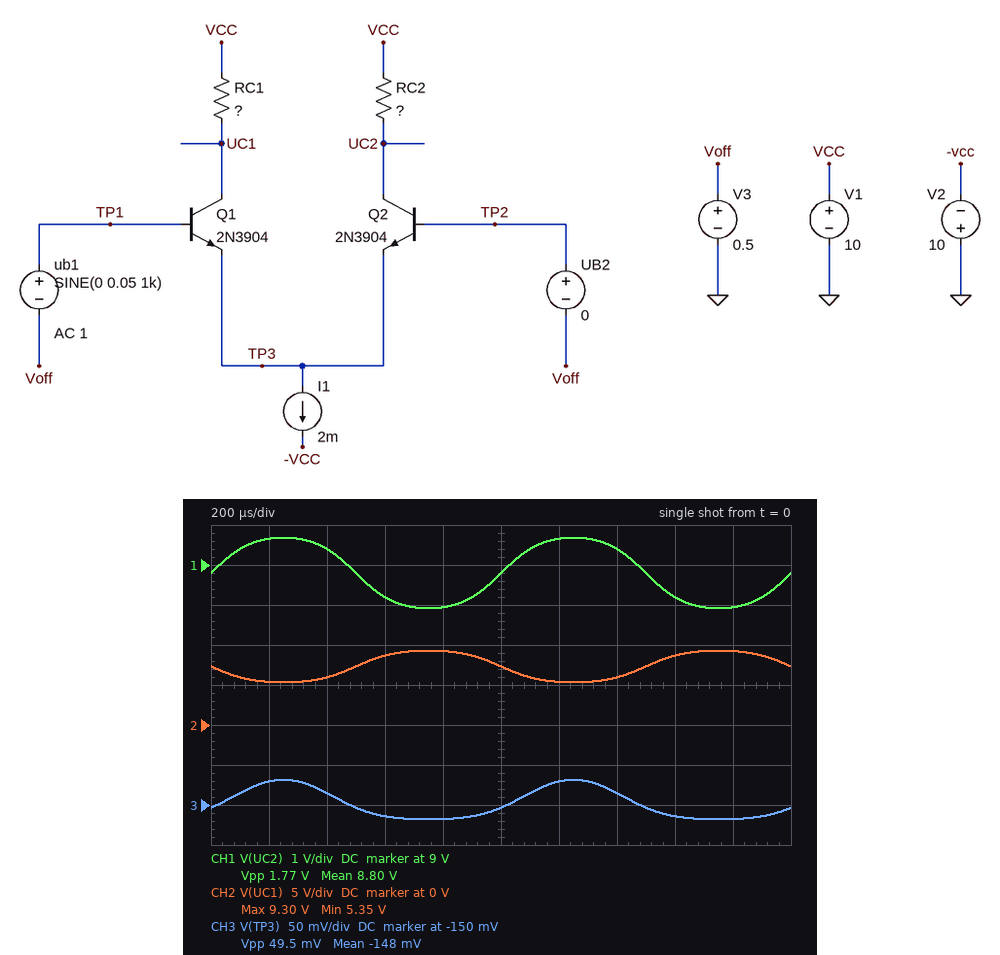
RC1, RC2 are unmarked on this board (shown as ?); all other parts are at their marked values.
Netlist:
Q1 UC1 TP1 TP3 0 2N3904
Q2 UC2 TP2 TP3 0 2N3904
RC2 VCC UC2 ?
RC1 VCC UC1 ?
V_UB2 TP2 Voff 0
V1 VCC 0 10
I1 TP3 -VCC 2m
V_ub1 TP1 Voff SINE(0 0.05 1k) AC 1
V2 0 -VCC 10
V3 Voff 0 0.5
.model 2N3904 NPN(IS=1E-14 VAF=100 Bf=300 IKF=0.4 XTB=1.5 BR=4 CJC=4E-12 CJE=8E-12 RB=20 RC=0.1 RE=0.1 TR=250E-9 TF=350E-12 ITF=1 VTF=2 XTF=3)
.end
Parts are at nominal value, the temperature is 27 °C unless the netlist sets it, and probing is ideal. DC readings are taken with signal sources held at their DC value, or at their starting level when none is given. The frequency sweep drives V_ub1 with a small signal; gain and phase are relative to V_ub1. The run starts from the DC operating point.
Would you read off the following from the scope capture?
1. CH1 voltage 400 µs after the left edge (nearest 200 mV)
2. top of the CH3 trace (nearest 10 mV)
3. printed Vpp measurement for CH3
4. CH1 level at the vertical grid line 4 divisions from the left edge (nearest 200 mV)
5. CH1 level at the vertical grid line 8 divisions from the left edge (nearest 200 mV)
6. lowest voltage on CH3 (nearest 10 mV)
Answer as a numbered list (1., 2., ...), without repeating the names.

1. 9.4 V
2. -120 mV
3. 49.5 mV
4. 8.0 V
5. 8.2 V
6. -170 mV
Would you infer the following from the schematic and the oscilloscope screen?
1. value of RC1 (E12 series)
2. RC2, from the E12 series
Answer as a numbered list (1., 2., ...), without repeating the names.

1. 2.7 kΩ
2. 1.2 kΩ
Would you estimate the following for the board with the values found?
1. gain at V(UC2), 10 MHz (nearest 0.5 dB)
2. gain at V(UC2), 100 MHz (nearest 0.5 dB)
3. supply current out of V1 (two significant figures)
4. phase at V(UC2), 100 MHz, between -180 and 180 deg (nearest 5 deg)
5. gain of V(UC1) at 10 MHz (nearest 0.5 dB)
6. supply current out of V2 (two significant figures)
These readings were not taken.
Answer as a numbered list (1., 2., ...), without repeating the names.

1. 26.5 dB
2. 18.0 dB
3. 2.0 mA
4. -75 deg
5. 33.0 dB
6. 2.0 mA
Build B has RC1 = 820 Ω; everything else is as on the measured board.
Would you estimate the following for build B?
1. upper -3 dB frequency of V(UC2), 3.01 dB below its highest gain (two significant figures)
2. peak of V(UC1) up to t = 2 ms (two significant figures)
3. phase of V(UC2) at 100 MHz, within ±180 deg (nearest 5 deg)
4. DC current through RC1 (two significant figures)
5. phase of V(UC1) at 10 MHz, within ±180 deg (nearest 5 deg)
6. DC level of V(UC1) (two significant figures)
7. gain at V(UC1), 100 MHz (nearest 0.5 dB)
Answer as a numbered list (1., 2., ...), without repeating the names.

1. 43 MHz
2. 9.8 V
3. -80 deg
4. 1.0 mA
5. 170 deg
6. 9.2 V
7. 17.5 dB
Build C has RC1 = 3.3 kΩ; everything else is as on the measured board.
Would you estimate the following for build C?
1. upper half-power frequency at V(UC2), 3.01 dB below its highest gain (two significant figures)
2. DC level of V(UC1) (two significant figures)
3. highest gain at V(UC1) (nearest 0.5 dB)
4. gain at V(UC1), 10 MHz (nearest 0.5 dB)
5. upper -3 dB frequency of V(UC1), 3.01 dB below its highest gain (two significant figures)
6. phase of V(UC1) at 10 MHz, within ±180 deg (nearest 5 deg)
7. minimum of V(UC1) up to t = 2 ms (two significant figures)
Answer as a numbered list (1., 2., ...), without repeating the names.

1. 29 MHz
2. 6.7 V
3. 36.0 dB
4. 34.5 dB
5. 17 MHz
6. 145 deg
7. 4.3 V
